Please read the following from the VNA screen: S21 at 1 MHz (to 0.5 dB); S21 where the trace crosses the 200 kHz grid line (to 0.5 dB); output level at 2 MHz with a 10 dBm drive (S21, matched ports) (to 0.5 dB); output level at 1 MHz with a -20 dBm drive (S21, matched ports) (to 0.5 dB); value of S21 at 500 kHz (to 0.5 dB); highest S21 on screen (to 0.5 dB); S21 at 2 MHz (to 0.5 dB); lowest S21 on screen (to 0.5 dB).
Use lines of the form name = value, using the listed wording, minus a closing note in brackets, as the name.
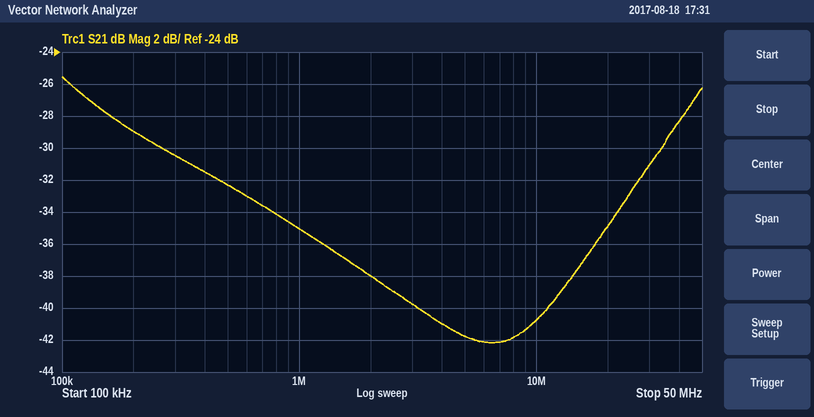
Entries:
S21 at 1 MHz = -35.0 dB
S21 where the trace crosses the 200 kHz grid line = -29.0 dB
output level at 2 MHz with a 10 dBm drive (S21, matched ports) = -28.0 dBm
output level at 1 MHz with a -20 dBm drive (S21, matched ports) = -55.0 dBm
value of S21 at 500 kHz = -32.5 dB
highest S21 on screen = -25.5 dB
S21 at 2 MHz = -38.0 dB
lowest S21 on screen = -42.0 dB
